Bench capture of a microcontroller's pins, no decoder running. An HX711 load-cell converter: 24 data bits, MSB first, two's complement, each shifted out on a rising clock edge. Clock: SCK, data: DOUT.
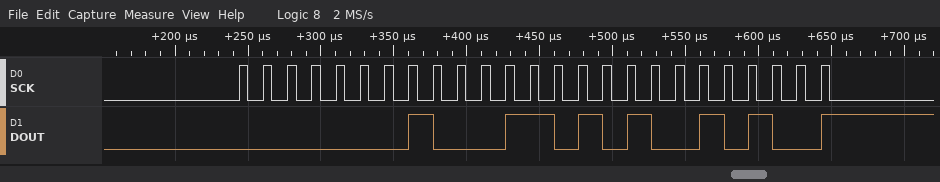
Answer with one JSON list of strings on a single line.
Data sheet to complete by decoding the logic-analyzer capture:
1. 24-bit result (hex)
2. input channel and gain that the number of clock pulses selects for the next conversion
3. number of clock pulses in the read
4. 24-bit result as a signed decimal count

["0x011A94", "channel A, gain 128", "25", "72340"]
